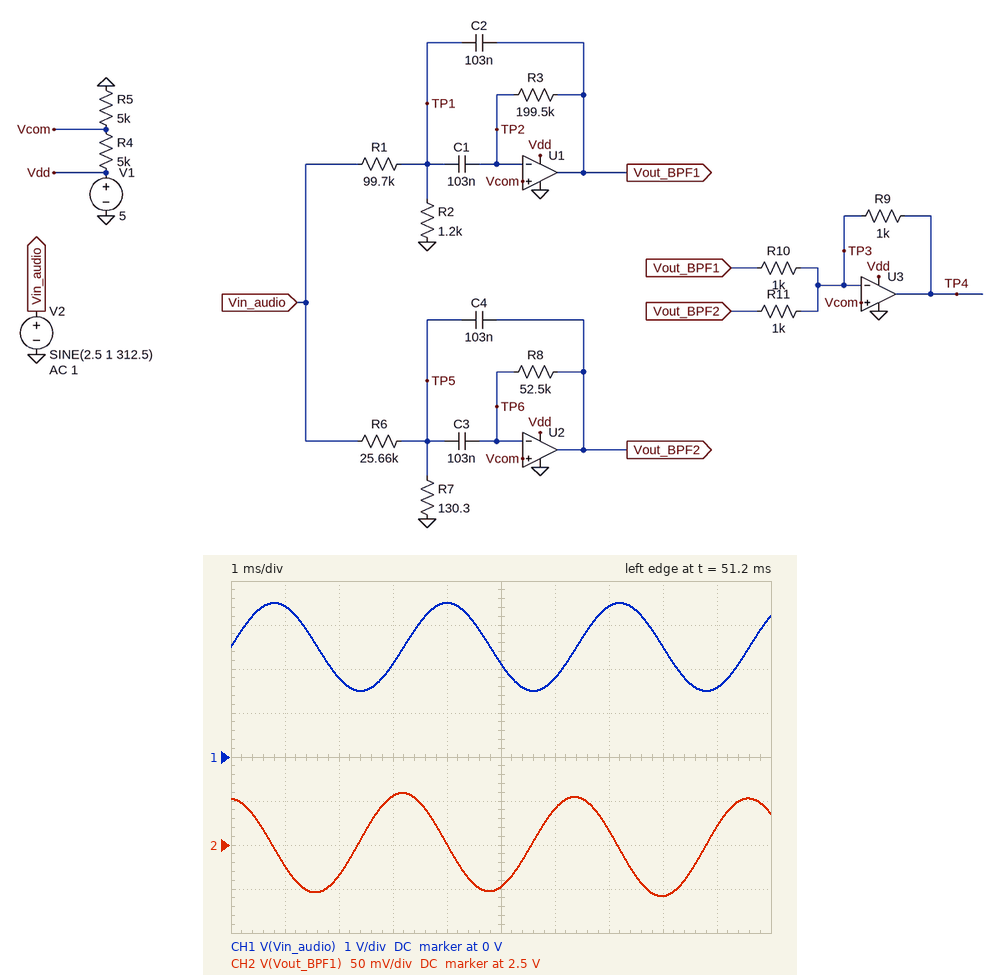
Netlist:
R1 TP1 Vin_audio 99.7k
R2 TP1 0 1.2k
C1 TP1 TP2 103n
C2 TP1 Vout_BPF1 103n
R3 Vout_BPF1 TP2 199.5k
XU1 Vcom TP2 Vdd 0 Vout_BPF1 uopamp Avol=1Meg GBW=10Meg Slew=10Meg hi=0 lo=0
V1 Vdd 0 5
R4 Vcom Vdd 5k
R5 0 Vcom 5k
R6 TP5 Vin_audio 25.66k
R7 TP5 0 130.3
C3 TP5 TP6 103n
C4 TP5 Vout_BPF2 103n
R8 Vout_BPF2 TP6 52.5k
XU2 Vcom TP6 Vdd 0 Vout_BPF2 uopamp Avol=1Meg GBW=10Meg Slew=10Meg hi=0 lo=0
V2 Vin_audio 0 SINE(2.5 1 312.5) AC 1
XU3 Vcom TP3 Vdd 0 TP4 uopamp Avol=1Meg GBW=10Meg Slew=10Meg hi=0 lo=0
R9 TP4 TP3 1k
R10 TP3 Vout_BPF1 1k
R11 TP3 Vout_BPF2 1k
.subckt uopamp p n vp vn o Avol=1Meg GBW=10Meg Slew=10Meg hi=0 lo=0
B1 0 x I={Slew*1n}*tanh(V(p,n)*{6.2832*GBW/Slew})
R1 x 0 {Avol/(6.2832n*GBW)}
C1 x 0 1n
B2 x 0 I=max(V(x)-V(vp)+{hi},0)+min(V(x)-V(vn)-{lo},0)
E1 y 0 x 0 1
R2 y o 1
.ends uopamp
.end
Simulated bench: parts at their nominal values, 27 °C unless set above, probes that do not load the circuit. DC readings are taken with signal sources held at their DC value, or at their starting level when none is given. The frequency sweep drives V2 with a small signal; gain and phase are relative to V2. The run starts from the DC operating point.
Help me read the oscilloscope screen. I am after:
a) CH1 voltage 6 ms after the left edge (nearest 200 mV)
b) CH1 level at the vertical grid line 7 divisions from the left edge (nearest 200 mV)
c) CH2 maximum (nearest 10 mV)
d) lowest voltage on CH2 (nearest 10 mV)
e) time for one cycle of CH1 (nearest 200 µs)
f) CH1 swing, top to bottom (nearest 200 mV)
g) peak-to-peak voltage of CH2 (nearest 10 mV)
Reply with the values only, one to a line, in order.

1.8 V
3.4 V
2.56 V
2.44 V
3.2 ms
2.0 V
120 mV
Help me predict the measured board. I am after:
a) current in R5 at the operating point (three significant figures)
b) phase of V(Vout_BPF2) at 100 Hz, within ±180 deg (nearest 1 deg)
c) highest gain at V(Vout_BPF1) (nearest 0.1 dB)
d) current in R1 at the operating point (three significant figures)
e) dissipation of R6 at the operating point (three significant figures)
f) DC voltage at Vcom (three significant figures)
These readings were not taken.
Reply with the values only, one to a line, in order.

500 µA
-91 deg
0 dB
24.8 µA
241 µW
2.50 V
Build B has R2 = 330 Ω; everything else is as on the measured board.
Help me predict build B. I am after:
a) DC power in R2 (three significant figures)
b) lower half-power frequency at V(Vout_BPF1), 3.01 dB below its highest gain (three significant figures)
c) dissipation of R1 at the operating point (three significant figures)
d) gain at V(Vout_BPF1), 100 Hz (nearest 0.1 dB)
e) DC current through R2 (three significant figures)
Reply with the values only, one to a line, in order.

206 nW
183 Hz
62.3 µW
-24.6 dB
25.0 µA
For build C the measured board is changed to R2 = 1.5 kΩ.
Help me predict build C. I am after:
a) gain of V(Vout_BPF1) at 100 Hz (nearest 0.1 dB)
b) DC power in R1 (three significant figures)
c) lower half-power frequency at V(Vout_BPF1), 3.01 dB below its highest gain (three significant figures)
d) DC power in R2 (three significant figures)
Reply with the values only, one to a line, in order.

-4.0 dB
60.8 µW
82.6 Hz
915 nW
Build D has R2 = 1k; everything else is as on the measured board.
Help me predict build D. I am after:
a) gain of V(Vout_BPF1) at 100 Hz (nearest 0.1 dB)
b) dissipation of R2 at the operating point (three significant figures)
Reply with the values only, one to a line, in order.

-4.5 dB
616 nW
